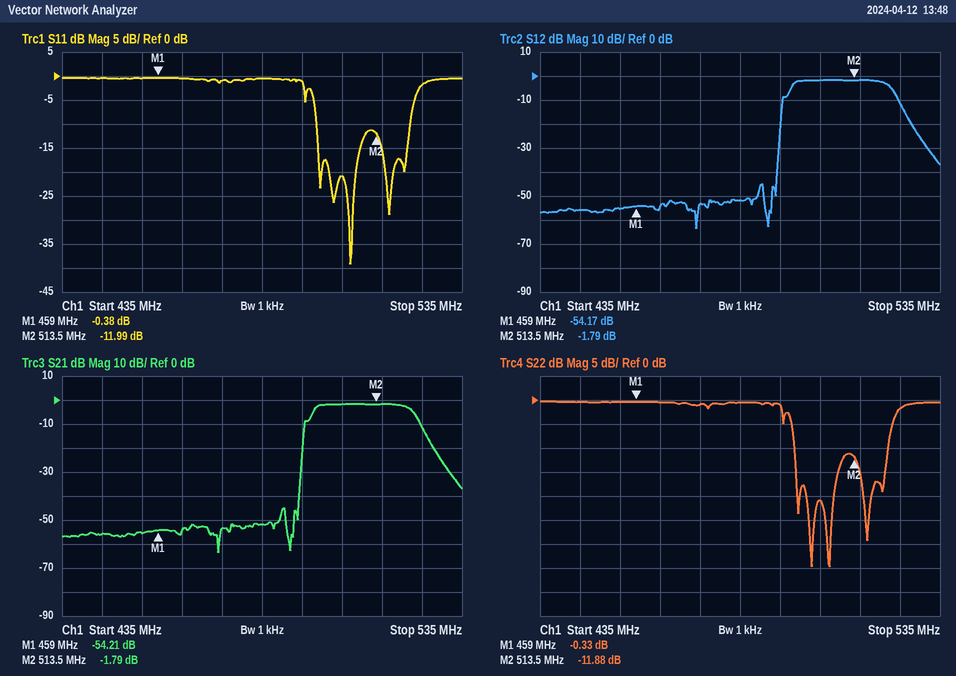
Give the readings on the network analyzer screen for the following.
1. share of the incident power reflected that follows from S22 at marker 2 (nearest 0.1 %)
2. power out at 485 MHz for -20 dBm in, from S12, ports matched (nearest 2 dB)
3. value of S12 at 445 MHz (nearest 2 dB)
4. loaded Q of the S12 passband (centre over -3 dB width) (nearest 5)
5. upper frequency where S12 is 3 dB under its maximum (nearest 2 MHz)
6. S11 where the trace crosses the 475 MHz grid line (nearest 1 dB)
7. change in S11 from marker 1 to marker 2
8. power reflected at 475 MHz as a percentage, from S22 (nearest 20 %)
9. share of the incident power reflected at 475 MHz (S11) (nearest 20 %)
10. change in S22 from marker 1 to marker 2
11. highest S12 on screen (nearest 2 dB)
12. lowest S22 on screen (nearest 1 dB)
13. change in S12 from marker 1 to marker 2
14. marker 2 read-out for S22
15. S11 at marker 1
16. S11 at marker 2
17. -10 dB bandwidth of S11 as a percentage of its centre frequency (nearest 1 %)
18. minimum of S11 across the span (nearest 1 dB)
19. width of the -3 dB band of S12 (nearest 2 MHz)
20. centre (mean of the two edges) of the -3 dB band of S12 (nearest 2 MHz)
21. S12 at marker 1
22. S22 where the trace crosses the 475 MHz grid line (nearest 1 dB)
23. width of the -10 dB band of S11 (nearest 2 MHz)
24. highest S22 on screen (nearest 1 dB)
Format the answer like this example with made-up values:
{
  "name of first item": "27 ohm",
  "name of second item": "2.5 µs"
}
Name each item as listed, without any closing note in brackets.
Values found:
{
  "share of the incident power reflected that follows from S22 at marker 2": "6.5 %",
  "power out at 485 MHz for -20 dBm in, from S12, ports matched": "-72 dBm",
  "value of S12 at 445 MHz": "-56 dB",
  "loaded Q of the S12 passband (centre over -3 dB width)": "20",
  "upper frequency where S12 is 3 dB under its maximum": "522 MHz",
  "S11 where the trace crosses the 475 MHz grid line": "-1 dB",
  "change in S11 from marker 1 to marker 2": "-11.61 dB",
  "power reflected at 475 MHz as a percentage, from S22": "80 %",
  "share of the incident power reflected at 475 MHz (S11)": "80 %",
  "change in S22 from marker 1 to marker 2": "-11.55 dB",
  "highest S12 on screen": "-2 dB",
  "lowest S22 on screen": "-35 dB",
  "change in S12 from marker 1 to marker 2": "52.38 dB",
  "marker 2 read-out for S22": "-11.88 dB",
  "S11 at marker 1": "-0.38 dB",
  "S11 at marker 2": "-11.99 dB",
  "-10 dB bandwidth of S11 as a percentage of its centre frequency": "5 %",
  "minimum of S11 across the span": "-39 dB",
  "width of the -3 dB band of S12": "24 MHz",
  "centre (mean of the two edges) of the -3 dB band of S12": "510 MHz",
  "S12 at marker 1": "-54.17 dB",
  "S22 where the trace crosses the 475 MHz grid line": "-1 dB",
  "width of the -10 dB band of S11": "24 MHz",
  "highest S22 on screen": "0 dB"
}
